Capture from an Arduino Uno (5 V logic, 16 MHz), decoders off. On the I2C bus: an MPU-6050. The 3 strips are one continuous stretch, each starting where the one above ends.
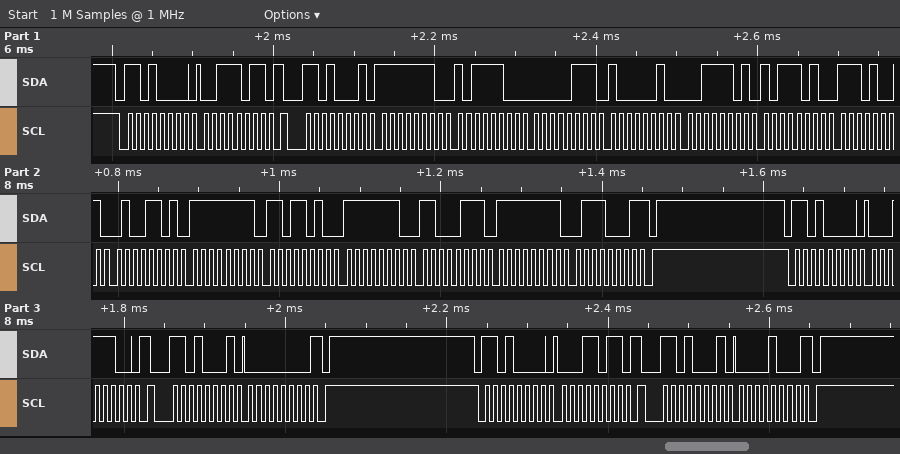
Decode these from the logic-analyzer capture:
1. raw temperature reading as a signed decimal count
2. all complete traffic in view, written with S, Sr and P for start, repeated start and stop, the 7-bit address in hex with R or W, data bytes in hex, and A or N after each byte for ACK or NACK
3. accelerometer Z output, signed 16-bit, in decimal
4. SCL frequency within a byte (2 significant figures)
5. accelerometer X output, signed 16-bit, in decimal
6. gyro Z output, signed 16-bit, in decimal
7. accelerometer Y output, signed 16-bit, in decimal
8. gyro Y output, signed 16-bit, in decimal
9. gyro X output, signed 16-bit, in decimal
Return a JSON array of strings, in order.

["-5811", "S 68W A 3B A Sr 68R A FE A BC A 07 A 82 A 3D A BA A E9 A 4D A FF A DA A FE A C7 A FF A 71 N P S 68W A 1C A Sr 68R A 00 N P S 68W A 1B A Sr 68R A 08 N P", "15802", "100 kHz", "-324", "-143", "1922", "-313", "-38"]
